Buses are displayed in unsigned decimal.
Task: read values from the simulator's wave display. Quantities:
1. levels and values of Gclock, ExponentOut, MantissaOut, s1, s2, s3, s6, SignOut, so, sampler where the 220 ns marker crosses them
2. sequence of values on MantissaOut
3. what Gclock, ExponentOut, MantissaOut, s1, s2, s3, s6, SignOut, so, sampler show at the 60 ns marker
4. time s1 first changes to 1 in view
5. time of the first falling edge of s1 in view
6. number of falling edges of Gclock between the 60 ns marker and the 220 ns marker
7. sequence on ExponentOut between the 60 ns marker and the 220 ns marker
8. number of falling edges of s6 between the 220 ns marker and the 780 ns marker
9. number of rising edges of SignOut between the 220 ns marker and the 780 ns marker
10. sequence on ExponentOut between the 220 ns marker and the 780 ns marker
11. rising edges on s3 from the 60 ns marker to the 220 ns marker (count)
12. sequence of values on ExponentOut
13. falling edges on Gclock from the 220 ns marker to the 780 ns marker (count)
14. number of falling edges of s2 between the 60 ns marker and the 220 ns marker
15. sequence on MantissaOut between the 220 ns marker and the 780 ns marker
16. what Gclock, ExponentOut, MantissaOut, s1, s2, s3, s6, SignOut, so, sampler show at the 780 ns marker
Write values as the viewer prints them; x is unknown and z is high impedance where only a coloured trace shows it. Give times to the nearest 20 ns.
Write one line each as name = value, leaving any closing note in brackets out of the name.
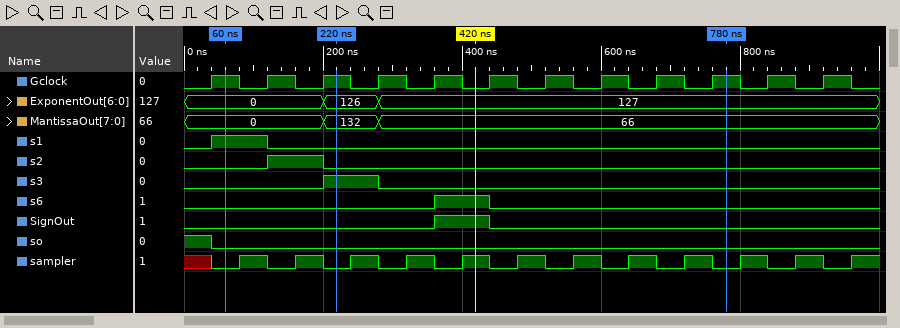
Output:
levels and values of Gclock, ExponentOut, MantissaOut, s1, s2, s3, s6, SignOut, so, sampler where the 220 ns marker crosses them = Gclock=1, ExponentOut=126, MantissaOut=132, s1=0, s2=0, s3=1, s6=0, SignOut=0, so=0, sampler=0
sequence of values on MantissaOut = 0, 132, 66
what Gclock, ExponentOut, MantissaOut, s1, s2, s3, s6, SignOut, so, sampler show at the 60 ns marker = Gclock=1, ExponentOut=0, MantissaOut=0, s1=1, s2=0, s3=0, s6=0, SignOut=0, so=0, sampler=0
time s1 first changes to 1 in view = 40 ns
time of the first falling edge of s1 in view = 120 ns
number of falling edges of Gclock between the 60 ns marker and the 220 ns marker = 2
sequence on ExponentOut between the 60 ns marker and the 220 ns marker = 0, 126
number of falling edges of s6 between the 220 ns marker and the 780 ns marker = 1
number of rising edges of SignOut between the 220 ns marker and the 780 ns marker = 1
sequence on ExponentOut between the 220 ns marker and the 780 ns marker = 126, 127
rising edges on s3 from the 60 ns marker to the 220 ns marker = 1
sequence of values on ExponentOut = 0, 126, 127
falling edges on Gclock from the 220 ns marker to the 780 ns marker = 7
number of falling edges of s2 between the 60 ns marker and the 220 ns marker = 1
sequence on MantissaOut between the 220 ns marker and the 780 ns marker = 132, 66
what Gclock, ExponentOut, MantissaOut, s1, s2, s3, s6, SignOut, so, sampler show at the 780 ns marker = Gclock=1, ExponentOut=127, MantissaOut=66, s1=0, s2=0, s3=0, s6=0, SignOut=0, so=0, sampler=0
